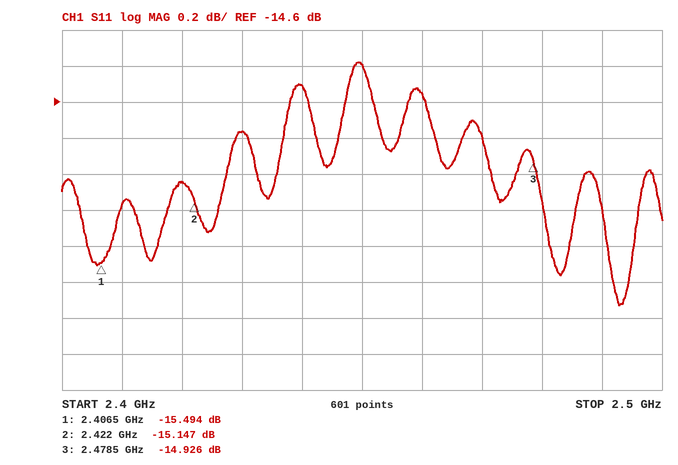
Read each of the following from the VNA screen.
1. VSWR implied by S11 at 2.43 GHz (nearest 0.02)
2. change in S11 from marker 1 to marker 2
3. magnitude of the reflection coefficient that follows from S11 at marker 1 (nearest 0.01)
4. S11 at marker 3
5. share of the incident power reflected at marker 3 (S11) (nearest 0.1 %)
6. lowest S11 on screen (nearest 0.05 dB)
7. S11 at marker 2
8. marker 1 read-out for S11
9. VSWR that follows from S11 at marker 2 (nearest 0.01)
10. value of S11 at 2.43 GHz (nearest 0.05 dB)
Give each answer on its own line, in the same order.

1.44
0.347 dB
0.17
-14.926 dB
3.2 %
-15.75 dB
-15.147 dB
-15.494 dB
1.42
-14.75 dB
